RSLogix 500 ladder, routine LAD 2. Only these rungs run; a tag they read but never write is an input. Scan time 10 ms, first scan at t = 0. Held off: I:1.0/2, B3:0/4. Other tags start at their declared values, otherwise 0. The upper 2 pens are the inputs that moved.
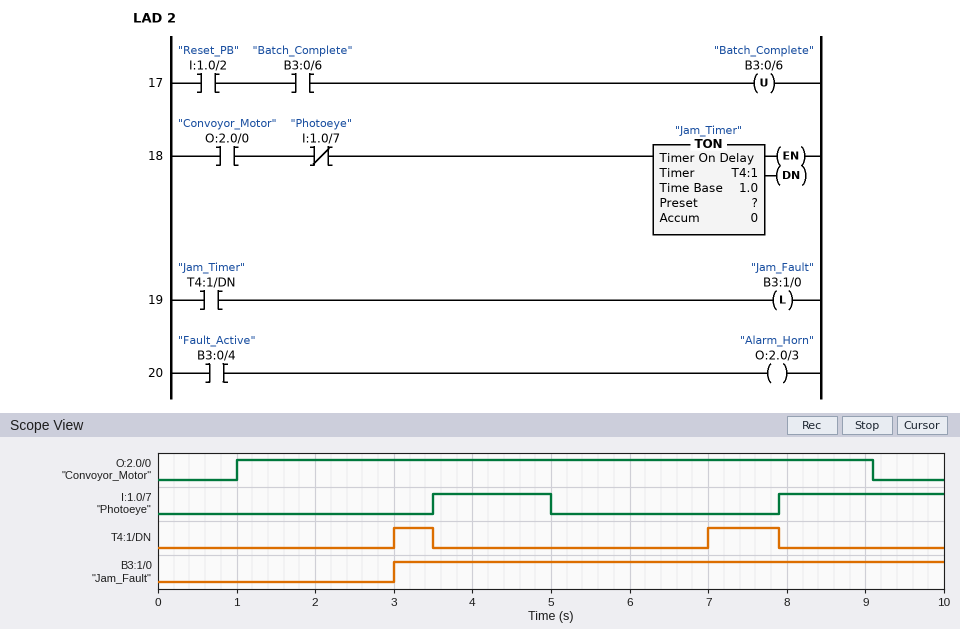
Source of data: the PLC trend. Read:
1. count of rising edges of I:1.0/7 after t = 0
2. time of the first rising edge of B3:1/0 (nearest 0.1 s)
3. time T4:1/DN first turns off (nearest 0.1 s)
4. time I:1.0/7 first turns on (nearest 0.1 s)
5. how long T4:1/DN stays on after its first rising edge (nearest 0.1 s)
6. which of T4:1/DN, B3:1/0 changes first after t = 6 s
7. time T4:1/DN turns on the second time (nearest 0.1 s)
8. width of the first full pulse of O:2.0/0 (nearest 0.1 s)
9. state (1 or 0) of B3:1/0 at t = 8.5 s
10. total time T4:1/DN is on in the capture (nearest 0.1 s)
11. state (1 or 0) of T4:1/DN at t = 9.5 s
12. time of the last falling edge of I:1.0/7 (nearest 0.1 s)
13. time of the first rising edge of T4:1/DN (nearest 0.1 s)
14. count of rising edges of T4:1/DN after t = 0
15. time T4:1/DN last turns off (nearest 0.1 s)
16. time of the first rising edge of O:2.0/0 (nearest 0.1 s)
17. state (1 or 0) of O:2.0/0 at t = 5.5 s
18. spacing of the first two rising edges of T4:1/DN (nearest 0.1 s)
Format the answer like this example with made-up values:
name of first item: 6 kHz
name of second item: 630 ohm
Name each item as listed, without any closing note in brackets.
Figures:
count of rising edges of I:1.0/7 after t = 0: 2
time of the first rising edge of B3:1/0: 3.0 s
time T4:1/DN first turns off: 3.5 s
time I:1.0/7 first turns on: 3.5 s
how long T4:1/DN stays on after its first rising edge: 0.5 s
which of T4:1/DN, B3:1/0 changes first after t = 6 s: T4:1/DN
time T4:1/DN turns on the second time: 7.0 s
width of the first full pulse of O:2.0/0: 8.1 s
state (1 or 0) of B3:1/0 at t = 8.5 s: 1
total time T4:1/DN is on in the capture: 1.4 s
state (1 or 0) of T4:1/DN at t = 9.5 s: 0
time of the last falling edge of I:1.0/7: 5.0 s
time of the first rising edge of T4:1/DN: 3.0 s
count of rising edges of T4:1/DN after t = 0: 2
time T4:1/DN last turns off: 7.9 s
time of the first rising edge of O:2.0/0: 1.0 s
state (1 or 0) of O:2.0/0 at t = 5.5 s: 1
spacing of the first two rising edges of T4:1/DN: 4.0 s
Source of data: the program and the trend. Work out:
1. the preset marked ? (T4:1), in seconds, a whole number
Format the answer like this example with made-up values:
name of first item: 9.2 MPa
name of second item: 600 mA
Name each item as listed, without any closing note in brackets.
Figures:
the preset marked ? (T4:1), in seconds, a whole number: 2 s
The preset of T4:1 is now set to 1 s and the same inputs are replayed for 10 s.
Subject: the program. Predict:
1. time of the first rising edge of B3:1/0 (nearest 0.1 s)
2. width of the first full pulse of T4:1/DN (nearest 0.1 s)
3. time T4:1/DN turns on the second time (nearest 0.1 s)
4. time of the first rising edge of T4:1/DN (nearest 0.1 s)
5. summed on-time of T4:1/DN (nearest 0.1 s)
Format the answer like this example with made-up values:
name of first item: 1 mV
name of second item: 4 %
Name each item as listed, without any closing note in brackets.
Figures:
time of the first rising edge of B3:1/0: 2.0 s
width of the first full pulse of T4:1/DN: 1.5 s
time T4:1/DN turns on the second time: 6.0 s
time of the first rising edge of T4:1/DN: 2.0 s
summed on-time of T4:1/DN: 3.4 s
